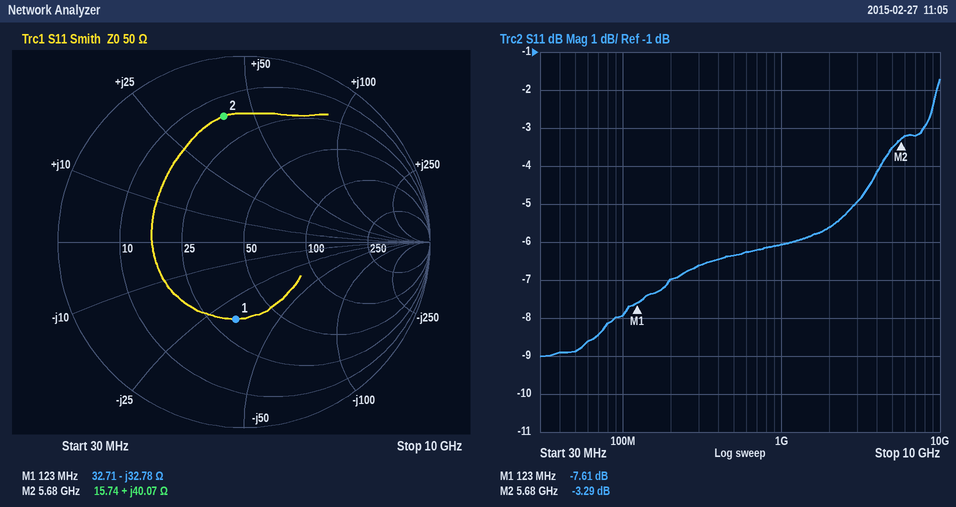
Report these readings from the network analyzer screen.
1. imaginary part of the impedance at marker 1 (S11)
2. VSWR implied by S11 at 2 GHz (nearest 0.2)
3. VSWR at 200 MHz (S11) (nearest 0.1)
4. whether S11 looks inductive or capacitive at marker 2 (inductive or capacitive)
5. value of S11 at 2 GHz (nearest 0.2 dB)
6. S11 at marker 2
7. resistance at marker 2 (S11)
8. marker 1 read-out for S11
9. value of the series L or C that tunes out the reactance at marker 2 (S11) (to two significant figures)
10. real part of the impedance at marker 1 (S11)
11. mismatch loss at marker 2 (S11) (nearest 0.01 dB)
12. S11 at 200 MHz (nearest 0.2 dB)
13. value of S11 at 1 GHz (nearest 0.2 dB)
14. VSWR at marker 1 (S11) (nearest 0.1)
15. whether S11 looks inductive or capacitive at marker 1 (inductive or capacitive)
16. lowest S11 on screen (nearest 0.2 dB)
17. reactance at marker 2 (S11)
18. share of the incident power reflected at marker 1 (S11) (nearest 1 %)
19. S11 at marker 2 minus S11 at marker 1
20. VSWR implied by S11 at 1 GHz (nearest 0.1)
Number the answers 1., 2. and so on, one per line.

1. -32.78 Ω
2. 3.2
3. 2.6
4. inductive
5. -5.6 dB
6. -3.29 dB
7. 15.74 Ω
8. -7.61 dB
9. 700 fF
10. 32.71 Ω
11. 2.75 dB
12. -7.0 dB
13. -6.0 dB
14. 2.4
15. capacitive
16. -9.0 dB
17. +40.07 Ω
18. 17 %
19. 4.32 dB
20. 3.0
